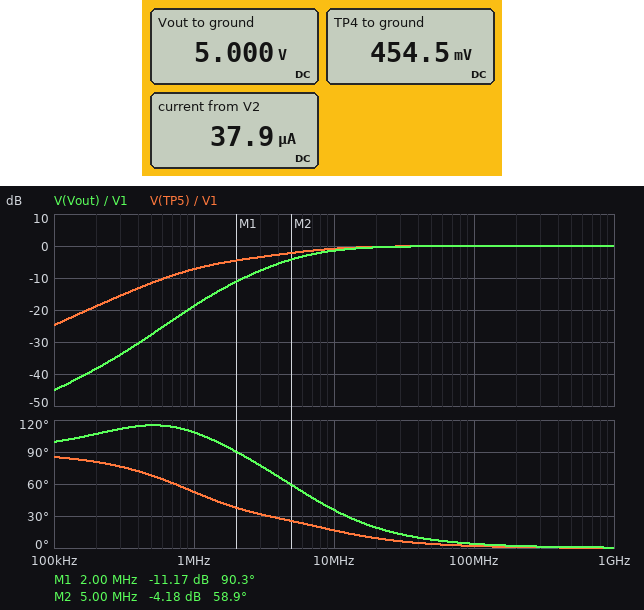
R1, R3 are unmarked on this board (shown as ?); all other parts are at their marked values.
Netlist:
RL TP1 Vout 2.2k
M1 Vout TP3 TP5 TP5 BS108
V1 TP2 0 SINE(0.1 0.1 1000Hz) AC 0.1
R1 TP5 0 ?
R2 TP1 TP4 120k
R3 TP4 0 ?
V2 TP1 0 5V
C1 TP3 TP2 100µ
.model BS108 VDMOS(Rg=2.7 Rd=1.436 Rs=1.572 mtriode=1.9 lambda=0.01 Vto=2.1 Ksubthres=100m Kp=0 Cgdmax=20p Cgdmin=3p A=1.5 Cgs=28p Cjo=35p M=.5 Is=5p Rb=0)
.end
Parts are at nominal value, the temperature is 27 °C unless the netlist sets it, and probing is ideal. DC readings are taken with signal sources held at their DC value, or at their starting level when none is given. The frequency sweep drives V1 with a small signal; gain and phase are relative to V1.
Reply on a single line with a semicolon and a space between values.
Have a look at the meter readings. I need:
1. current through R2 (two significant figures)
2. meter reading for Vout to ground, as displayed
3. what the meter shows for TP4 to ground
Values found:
38 µA; 5.000 V; 454.5 mV
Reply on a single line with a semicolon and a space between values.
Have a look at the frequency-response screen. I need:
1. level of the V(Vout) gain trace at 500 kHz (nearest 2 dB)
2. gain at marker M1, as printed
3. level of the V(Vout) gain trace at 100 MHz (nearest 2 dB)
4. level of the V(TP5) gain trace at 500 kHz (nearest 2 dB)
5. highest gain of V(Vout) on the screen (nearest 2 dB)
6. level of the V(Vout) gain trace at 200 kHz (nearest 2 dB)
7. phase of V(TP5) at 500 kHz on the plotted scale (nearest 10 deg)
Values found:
-28 dB; -11.17 dB; 0 dB; -12 dB; 0 dB; -38 dB; 70 deg
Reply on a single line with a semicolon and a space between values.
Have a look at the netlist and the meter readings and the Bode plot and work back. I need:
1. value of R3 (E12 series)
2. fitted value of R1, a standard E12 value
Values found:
12 kΩ; 3.3 kΩ
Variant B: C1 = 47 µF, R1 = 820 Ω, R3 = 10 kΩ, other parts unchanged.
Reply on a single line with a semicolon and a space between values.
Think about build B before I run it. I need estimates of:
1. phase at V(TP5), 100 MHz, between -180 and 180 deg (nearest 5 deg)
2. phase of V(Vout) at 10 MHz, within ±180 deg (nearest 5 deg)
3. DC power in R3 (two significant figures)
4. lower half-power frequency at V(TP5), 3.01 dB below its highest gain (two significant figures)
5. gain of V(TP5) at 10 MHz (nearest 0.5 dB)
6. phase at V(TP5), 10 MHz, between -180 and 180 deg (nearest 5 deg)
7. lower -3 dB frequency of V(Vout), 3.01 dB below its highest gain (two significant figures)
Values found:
5 deg; 50 deg; 15 µW; 8.3 MHz; -2.5 dB; 35 deg; 9.6 MHz
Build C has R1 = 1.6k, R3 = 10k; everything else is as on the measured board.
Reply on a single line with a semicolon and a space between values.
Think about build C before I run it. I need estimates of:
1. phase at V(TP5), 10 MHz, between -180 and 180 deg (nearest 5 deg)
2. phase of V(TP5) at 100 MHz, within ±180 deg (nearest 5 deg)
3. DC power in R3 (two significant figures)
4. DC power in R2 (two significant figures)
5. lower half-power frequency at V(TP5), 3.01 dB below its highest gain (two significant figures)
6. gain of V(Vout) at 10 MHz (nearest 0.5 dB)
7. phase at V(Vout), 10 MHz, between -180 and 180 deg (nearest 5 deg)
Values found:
25 deg; 5 deg; 15 µW; 180 µW; 5.3 MHz; -2.0 dB; 40 deg
